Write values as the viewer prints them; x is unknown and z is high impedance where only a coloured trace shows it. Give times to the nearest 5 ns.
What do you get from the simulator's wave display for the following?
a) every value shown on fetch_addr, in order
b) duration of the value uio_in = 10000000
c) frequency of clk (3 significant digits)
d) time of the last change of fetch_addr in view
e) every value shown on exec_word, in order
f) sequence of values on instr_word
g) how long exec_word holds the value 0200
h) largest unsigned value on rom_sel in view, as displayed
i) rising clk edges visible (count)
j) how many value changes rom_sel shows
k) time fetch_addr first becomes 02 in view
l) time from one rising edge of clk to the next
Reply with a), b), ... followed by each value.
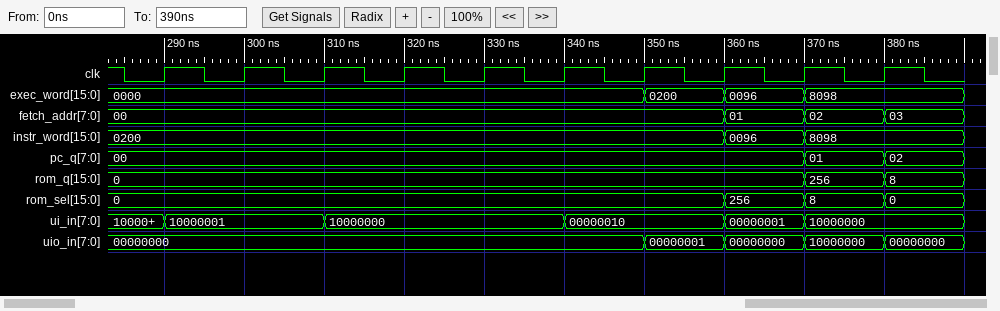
a) 00, 01, 02, 03
b) 10 ns
c) 100 MHz
d) 380 ns
e) 0000, 0200, 0096, 8098
f) 0200, 0096, 8098
g) 10 ns
h) 256
i) 10
j) 3
k) 370 ns
l) 10 ns
